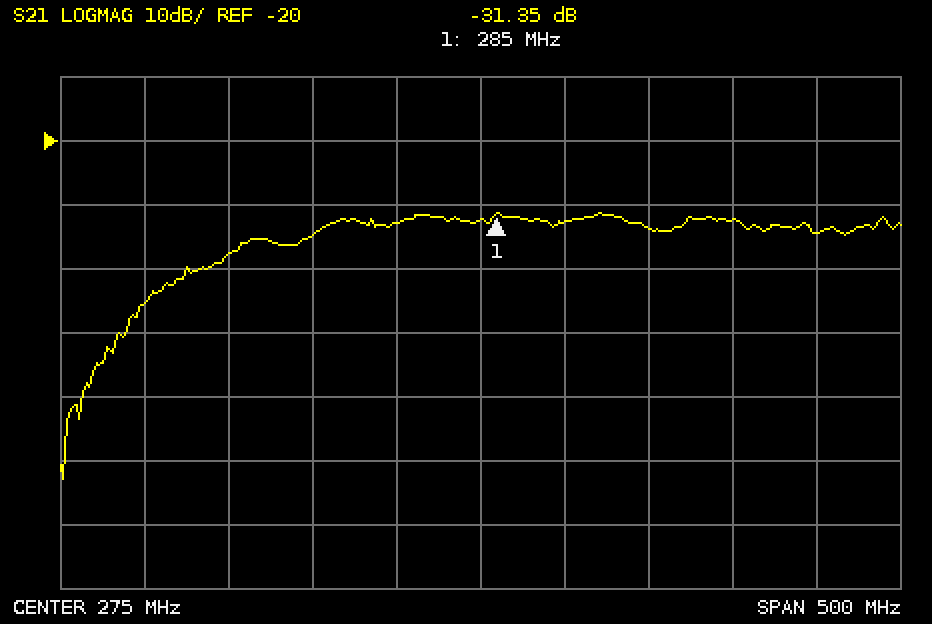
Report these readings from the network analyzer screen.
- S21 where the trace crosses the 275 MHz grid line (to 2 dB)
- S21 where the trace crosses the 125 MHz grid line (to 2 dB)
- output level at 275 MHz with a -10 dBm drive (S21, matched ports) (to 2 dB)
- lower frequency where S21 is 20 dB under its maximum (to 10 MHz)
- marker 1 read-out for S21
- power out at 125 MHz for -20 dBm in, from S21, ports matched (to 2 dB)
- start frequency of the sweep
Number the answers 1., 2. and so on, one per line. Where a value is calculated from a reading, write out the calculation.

1. -32 dB
2. -38 dB
3. -10 dBm + (-32 dB) = -42 dBm
4. 60 MHz
5. -31.35 dB
6. -20 dBm + (-38 dB) = -58 dBm
7. 25 MHz
